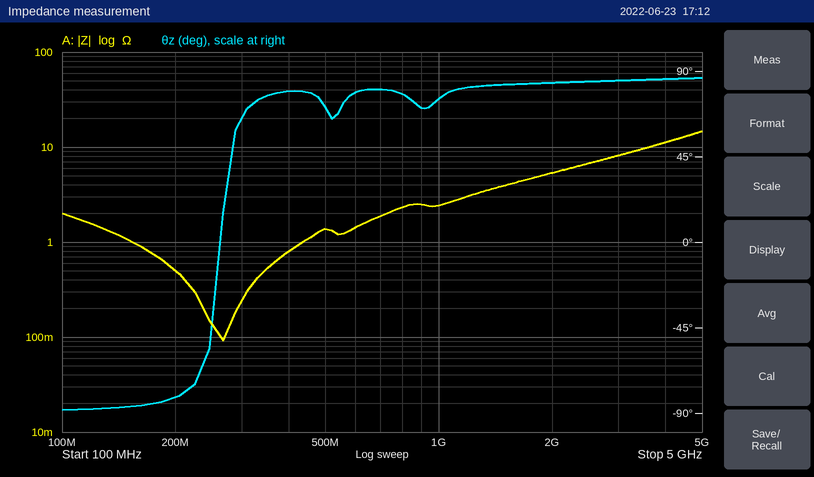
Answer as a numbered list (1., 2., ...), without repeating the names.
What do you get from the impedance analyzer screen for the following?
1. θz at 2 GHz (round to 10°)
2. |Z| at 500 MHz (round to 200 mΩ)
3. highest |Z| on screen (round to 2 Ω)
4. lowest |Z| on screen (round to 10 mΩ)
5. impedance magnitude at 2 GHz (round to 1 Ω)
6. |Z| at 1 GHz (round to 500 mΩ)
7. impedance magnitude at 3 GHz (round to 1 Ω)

1. 80°
2. 1.4 Ω
3. 14 Ω
4. 90 mΩ
5. 5 Ω
6. 2.5 Ω
7. 8 Ω
